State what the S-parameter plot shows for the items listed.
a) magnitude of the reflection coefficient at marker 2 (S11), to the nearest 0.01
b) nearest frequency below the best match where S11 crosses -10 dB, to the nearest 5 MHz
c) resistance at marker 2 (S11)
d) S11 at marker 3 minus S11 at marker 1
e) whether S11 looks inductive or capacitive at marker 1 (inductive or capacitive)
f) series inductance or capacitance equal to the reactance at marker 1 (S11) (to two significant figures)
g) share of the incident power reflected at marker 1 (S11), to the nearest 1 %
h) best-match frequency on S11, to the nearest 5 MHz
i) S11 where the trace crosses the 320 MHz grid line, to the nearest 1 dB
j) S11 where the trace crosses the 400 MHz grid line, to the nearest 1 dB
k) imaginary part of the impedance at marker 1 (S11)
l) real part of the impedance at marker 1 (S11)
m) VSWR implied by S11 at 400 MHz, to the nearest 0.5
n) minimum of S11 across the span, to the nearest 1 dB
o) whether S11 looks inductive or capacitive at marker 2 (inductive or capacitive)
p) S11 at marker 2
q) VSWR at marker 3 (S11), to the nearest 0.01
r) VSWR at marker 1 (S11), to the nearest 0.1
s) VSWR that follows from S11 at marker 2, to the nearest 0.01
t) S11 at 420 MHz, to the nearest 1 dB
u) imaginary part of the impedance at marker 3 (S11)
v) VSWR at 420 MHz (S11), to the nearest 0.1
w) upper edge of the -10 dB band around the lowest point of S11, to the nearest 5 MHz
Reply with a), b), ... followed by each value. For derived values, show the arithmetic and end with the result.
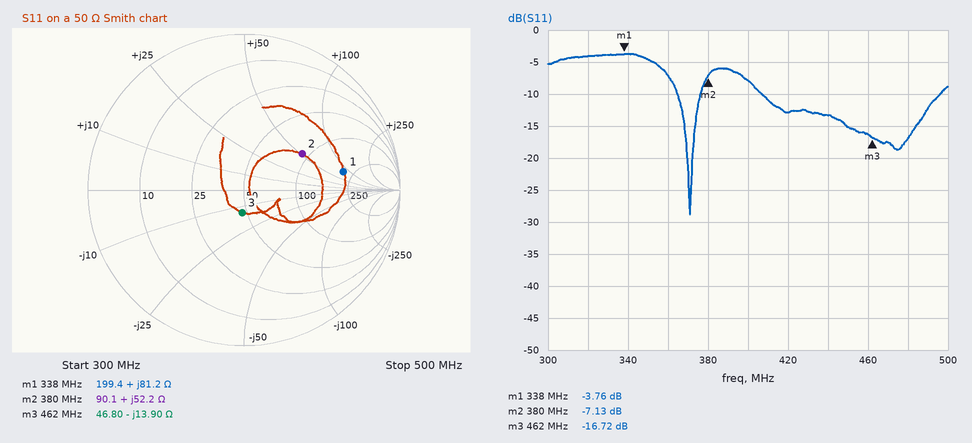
a) 0.44
b) 365 MHz
c) 90.1 Ω
d) -16.72 − (-3.76) = -12.96 dB
e) inductive
f) L = 81.2 Ω/(2π × 338 MHz) ≈ 38 nH
g) 10^(-3.76/10) ≈ 42 %
h) 370 MHz
i) -4 dB
j) -8 dB
k) +81.2 Ω
l) 199.4 Ω
m) |Γ| = 10^(-8/20) = 0.3981; VSWR = (1 + 0.3981)/(1 − 0.3981) ≈ 2.32, so 2.5 to the nearest 0.5
n) -29 dB
o) inductive
p) -7.13 dB
q) 1.34
r) 4.7
s) (1 + 0.4400)/(1 − 0.4400) ≈ 2.57
t) -13 dB
u) -13.90 Ω
v) |Γ| = 10^(-13/20) = 0.2239; VSWR = (1 + 0.2239)/(1 − 0.2239) ≈ 1.6
w) 375 MHz
